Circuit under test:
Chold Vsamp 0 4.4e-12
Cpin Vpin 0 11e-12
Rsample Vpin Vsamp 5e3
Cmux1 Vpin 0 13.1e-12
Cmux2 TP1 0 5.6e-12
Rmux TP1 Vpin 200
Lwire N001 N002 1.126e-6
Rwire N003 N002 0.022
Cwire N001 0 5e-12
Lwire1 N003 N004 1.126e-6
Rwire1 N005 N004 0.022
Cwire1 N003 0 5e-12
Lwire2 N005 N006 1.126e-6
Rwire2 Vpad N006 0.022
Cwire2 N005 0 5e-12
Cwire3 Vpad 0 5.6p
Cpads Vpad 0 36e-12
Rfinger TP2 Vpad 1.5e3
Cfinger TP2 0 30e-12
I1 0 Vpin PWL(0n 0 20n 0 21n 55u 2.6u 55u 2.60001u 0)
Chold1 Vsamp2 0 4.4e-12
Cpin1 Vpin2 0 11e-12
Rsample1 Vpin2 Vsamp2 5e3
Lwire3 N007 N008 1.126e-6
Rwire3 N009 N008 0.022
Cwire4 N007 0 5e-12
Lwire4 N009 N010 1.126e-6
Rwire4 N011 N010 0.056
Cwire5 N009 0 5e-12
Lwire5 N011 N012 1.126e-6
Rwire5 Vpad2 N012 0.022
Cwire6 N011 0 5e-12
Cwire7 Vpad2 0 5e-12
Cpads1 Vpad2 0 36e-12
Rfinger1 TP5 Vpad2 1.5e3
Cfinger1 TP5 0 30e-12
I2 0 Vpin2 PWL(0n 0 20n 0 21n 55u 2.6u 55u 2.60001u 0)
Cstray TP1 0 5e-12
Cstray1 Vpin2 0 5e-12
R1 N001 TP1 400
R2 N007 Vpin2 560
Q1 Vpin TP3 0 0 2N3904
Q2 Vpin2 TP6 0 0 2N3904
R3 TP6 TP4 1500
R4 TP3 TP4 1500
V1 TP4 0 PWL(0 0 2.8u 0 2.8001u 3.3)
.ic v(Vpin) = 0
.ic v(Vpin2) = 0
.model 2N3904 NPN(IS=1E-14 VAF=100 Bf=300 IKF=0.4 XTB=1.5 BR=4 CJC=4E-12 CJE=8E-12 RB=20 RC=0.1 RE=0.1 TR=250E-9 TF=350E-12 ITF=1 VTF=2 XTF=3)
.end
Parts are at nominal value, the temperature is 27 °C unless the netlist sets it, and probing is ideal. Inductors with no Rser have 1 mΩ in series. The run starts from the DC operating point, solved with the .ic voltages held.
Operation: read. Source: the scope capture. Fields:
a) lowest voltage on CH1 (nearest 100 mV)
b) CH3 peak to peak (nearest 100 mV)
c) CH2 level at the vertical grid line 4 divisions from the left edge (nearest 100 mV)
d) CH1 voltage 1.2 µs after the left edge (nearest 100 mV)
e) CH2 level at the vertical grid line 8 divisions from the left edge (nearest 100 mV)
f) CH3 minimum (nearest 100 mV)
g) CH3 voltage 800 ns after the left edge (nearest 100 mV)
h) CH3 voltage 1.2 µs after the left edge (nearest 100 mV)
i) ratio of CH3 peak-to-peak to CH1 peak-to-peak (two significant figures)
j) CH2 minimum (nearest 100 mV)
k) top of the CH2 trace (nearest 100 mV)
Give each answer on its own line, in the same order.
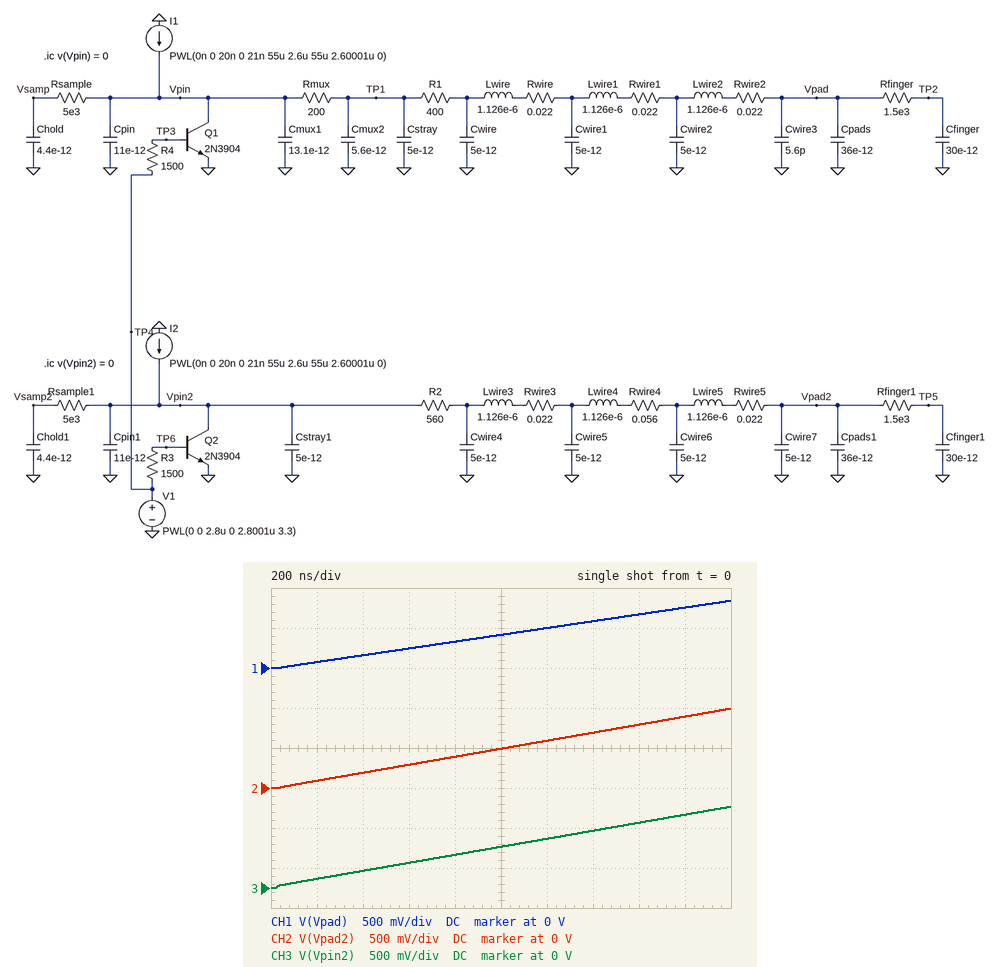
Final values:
0 V
1.0 V
400 mV
500 mV
800 mV
0 V
400 mV
600 mV
1.2
0 V
1.0 V
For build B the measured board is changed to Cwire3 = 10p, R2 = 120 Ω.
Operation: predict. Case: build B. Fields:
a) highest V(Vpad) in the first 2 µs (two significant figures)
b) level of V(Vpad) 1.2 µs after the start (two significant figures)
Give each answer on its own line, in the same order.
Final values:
810 mV
480 mV
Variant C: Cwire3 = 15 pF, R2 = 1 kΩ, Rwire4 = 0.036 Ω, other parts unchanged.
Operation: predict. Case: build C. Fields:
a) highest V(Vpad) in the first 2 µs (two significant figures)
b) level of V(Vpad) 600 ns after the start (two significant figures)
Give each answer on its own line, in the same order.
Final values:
780 mV
230 mV
